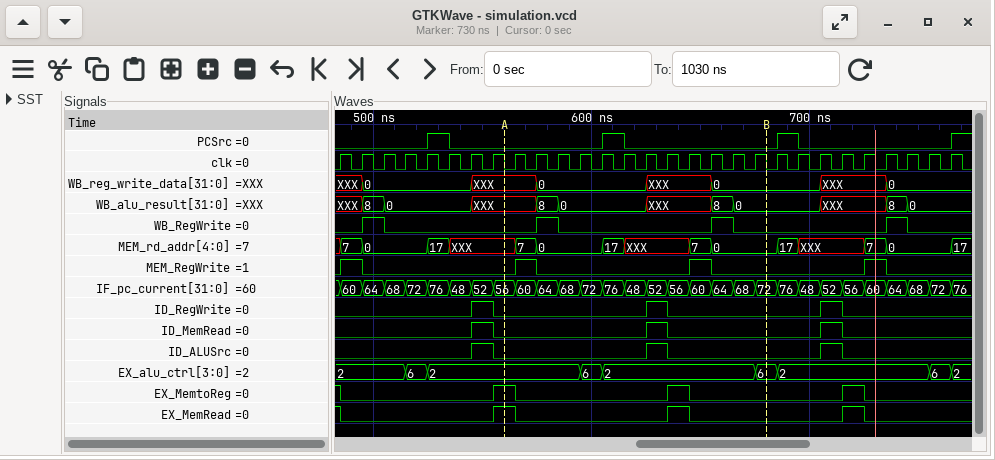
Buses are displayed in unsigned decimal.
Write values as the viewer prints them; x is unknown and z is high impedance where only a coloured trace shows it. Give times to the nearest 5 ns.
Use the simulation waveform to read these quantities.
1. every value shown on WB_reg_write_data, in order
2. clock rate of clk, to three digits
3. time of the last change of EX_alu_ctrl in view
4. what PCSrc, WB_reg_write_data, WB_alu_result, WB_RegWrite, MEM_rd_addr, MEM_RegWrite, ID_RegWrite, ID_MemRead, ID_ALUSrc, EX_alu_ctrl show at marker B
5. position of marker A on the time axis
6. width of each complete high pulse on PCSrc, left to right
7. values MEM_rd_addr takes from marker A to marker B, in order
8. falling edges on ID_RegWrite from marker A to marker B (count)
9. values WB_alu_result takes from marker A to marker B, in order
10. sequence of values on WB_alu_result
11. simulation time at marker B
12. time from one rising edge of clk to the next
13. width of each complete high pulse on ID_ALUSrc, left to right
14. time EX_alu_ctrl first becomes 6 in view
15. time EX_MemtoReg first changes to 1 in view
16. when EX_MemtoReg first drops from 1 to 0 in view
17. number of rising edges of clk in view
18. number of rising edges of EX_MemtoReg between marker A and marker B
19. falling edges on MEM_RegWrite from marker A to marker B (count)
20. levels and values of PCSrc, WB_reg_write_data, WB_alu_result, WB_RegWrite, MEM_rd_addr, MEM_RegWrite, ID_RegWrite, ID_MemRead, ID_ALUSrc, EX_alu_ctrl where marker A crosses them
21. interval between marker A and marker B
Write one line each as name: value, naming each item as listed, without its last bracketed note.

every value shown on WB_reg_write_data, in order: XXX, 0, XXX, 0, XXX, 0, XXX, 0
clock rate of clk, to three digits: 100 MHz
time of the last change of EX_alu_ctrl in view: 765 ns
what PCSrc, WB_reg_write_data, WB_alu_result, WB_RegWrite, MEM_rd_addr, MEM_RegWrite, ID_RegWrite, ID_MemRead, ID_ALUSrc, EX_alu_ctrl show at marker B: PCSrc=0, WB_reg_write_data=0, WB_alu_result=0, WB_RegWrite=0, MEM_rd_addr=0, MEM_RegWrite=0, ID_RegWrite=0, ID_MemRead=0, ID_ALUSrc=0, EX_alu_ctrl=6
position of marker A on the time axis: 560 ns
width of each complete high pulse on PCSrc, left to right: 10 ns, 10 ns, 10 ns
values MEM_rd_addr takes from marker A to marker B, in order: XXX, 7, 0, 17, XXX, 7, 0
falling edges on ID_RegWrite from marker A to marker B: 1
values WB_alu_result takes from marker A to marker B, in order: XXX, 8, 0, XXX, 8, 0
sequence of values on WB_alu_result: XXX, 8, 0, XXX, 8, 0, XXX, 8, 0, XXX, 8, 0
simulation time at marker B: 680 ns
time from one rising edge of clk to the next: 10 ns
width of each complete high pulse on ID_ALUSrc, left to right: 10 ns, 10 ns, 10 ns
time EX_alu_ctrl first becomes 6 in view: 515 ns
time EX_MemtoReg first changes to 1 in view: 555 ns
when EX_MemtoReg first drops from 1 to 0 in view: 485 ns
number of rising edges of clk in view: 29
number of rising edges of EX_MemtoReg between marker A and marker B: 1
falling edges on MEM_RegWrite from marker A to marker B: 2
levels and values of PCSrc, WB_reg_write_data, WB_alu_result, WB_RegWrite, MEM_rd_addr, MEM_RegWrite, ID_RegWrite, ID_MemRead, ID_ALUSrc, EX_alu_ctrl where marker A crosses them: PCSrc=0, WB_reg_write_data=XXX, WB_alu_result=XXX, WB_RegWrite=0, MEM_rd_addr=XXX, MEM_RegWrite=0, ID_RegWrite=0, ID_MemRead=0, ID_ALUSrc=0, EX_alu_ctrl=2
interval between marker A and marker B: 120 ns
